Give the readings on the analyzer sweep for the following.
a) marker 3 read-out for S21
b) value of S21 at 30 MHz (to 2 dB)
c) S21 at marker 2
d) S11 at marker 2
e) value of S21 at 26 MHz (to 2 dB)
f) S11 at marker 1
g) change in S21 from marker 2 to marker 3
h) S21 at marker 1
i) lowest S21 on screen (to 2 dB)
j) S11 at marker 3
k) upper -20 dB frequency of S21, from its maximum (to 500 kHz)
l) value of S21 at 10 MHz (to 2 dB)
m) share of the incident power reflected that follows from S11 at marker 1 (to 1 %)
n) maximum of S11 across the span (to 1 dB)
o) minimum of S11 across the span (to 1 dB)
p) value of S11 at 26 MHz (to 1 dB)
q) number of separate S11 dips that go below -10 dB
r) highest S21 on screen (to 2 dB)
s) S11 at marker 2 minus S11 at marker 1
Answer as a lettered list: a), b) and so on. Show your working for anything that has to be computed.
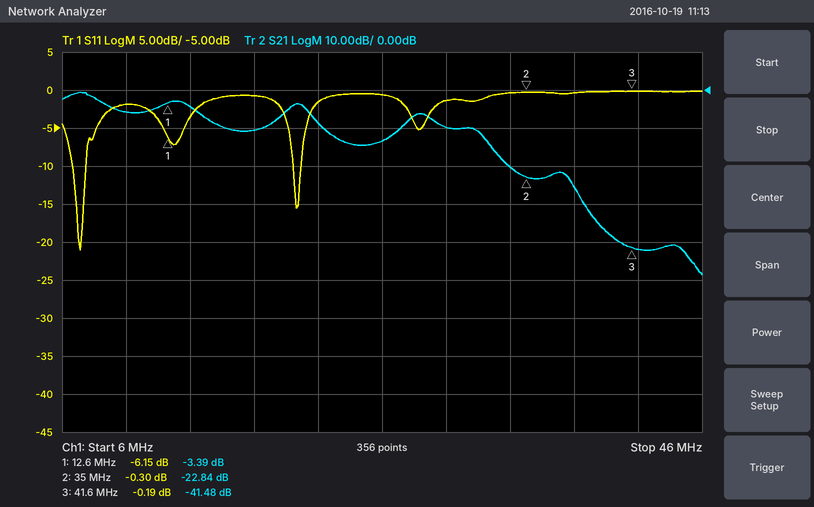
a) -41.48 dB
b) -10 dB
c) -22.84 dB
d) -0.30 dB
e) -14 dB
f) -6.15 dB
g) -41.48 − (-22.84) = -18.64 dB
h) -3.39 dB
i) -48 dB
j) -0.19 dB
k) 34.0 MHz
l) -6 dB
m) 10^(-6.15/10) ≈ 24 %
n) 0 dB
o) -21 dB
p) -1 dB
q) 2
r) 0 dB
s) -0.3 − (-6.15) = 5.85 dB
